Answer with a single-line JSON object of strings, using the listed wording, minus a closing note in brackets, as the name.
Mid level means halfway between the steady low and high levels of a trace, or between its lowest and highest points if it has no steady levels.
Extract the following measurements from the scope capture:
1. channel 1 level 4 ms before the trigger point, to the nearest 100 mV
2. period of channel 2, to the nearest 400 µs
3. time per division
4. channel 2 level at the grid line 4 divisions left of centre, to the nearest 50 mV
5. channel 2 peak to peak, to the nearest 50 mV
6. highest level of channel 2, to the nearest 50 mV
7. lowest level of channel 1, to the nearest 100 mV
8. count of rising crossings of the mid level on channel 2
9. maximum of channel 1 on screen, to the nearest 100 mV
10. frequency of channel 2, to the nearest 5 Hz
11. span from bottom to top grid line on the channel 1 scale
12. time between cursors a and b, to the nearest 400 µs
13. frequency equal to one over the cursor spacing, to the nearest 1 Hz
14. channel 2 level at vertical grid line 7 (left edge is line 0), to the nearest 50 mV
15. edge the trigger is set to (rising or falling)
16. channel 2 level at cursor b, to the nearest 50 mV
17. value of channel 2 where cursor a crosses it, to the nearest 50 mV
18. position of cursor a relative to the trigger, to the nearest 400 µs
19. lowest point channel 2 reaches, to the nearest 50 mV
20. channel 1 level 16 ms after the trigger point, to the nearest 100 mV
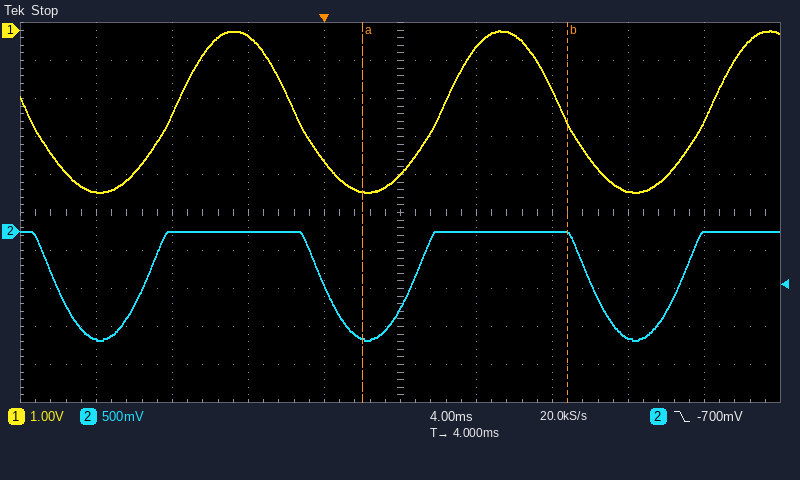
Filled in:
{"channel 1 level 4 ms before the trigger point, to the nearest 100 mV": "-200 mV", "period of channel 2, to the nearest 400 µs": "14.0 ms", "time per division": "4 ms", "channel 2 level at the grid line 4 divisions left of centre, to the nearest 50 mV": "-1.40 V", "channel 2 peak to peak, to the nearest 50 mV": "1.45 V", "highest level of channel 2, to the nearest 50 mV": "0 mV", "lowest level of channel 1, to the nearest 100 mV": "-4.3 V", "count of rising crossings of the mid level on channel 2": "3", "maximum of channel 1 on screen, to the nearest 100 mV": "0.0 V", "frequency of channel 2, to the nearest 5 Hz": "70 Hz", "span from bottom to top grid line on the channel 1 scale": "10 V", "time between cursors a and b, to the nearest 400 µs": "10.8 ms", "frequency equal to one over the cursor spacing, to the nearest 1 Hz": "93 Hz", "channel 2 level at vertical grid line 7 (left edge is line 0), to the nearest 50 mV": "0 mV", "edge the trigger is set to": "falling", "channel 2 level at cursor b, to the nearest 50 mV": "-50 mV", "value of channel 2 where cursor a crosses it, to the nearest 50 mV": "-1.40 V", "position of cursor a relative to the trigger, to the nearest 400 µs": "+2.0 ms", "lowest point channel 2 reaches, to the nearest 50 mV": "-1.45 V", "channel 1 level 16 ms after the trigger point, to the nearest 100 mV": "-4.2 V"}
